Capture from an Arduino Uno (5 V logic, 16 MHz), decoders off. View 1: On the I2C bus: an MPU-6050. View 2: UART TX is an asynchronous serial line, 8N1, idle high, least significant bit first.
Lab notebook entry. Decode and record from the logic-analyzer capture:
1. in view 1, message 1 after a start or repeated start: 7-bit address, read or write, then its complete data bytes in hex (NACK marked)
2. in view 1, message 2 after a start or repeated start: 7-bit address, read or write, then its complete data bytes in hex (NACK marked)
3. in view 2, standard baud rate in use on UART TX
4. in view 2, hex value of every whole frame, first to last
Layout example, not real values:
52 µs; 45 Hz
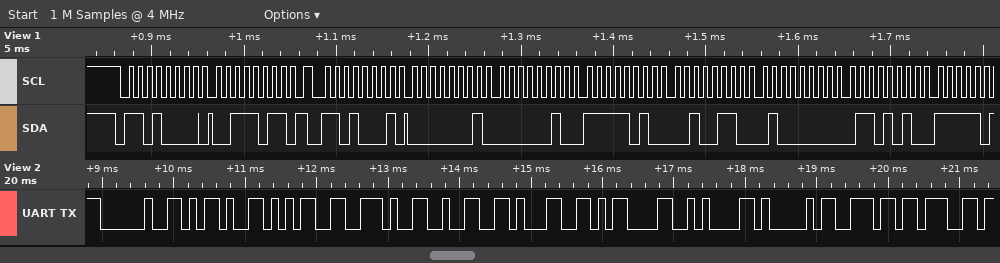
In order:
0x68 write: 3B; 0x68 read: 01 02 FA 26 40 6A; 9600 baud; 20 2D 35 2E 32 31 0D 0A 41 6E 67
